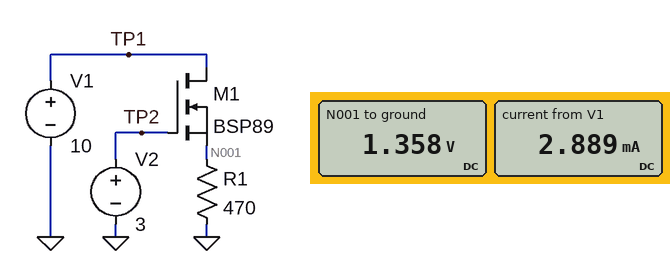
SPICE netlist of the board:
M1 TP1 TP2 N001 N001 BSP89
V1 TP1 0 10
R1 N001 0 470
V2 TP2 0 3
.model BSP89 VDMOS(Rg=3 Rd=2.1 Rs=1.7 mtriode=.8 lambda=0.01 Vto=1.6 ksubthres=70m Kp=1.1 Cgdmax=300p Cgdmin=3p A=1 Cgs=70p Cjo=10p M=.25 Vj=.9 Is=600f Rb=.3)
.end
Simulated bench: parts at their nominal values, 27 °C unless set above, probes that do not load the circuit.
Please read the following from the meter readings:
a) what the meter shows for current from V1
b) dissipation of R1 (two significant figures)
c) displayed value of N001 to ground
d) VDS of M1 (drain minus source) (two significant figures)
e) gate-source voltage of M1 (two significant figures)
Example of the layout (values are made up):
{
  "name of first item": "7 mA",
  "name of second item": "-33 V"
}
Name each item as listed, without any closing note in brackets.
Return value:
{
  "what the meter shows for current from V1": "2.889 mA",
  "dissipation of R1": "3.9 mW",
  "displayed value of N001 to ground": "1.358 V",
  "VDS of M1 (drain minus source)": "8.6 V",
  "gate-source voltage of M1": "1.6 V"
}
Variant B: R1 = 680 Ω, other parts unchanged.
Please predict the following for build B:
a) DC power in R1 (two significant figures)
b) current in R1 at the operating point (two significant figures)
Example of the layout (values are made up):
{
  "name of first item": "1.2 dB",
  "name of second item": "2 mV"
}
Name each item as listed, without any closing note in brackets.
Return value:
{
  "DC power in R1": "2.8 mW",
  "current in R1 at the operating point": "2.0 mA"
}
